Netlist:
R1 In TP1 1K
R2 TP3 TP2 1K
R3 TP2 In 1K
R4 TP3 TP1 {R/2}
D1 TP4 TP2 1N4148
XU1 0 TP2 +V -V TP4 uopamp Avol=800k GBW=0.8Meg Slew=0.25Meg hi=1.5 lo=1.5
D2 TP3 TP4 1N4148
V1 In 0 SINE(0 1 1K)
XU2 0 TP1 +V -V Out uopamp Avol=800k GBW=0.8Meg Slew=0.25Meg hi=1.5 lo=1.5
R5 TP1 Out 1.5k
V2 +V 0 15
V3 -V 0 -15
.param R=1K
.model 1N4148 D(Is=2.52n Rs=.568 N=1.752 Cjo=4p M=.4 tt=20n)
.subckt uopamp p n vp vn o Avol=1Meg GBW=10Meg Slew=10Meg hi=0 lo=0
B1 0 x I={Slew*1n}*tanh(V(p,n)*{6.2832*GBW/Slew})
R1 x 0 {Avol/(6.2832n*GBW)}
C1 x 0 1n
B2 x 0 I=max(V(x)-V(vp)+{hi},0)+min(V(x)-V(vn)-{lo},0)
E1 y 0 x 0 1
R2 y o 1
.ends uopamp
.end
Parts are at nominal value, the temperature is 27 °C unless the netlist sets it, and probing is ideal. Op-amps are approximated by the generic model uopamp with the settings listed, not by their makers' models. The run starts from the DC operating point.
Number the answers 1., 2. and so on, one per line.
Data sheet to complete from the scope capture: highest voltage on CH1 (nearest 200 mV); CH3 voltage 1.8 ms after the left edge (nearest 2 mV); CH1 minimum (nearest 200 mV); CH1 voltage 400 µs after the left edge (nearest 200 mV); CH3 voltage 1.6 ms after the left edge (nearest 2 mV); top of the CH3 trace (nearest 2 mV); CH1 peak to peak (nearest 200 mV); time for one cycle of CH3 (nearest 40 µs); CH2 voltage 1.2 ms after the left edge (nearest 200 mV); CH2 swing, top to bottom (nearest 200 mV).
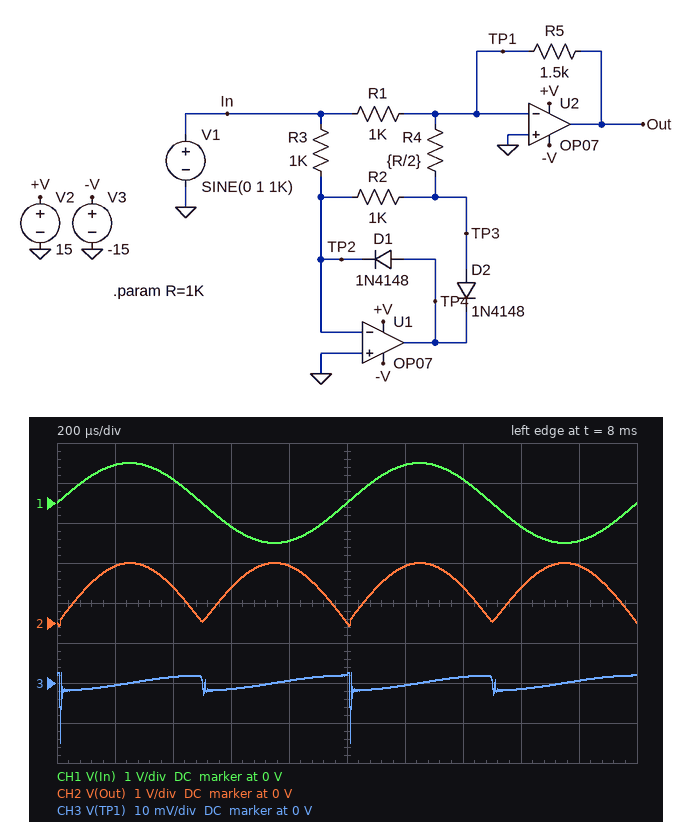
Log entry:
1. 1.0 V
2. 0 V
3. -1.0 V
4. 600 mV
5. -2 mV
6. 2 mV
7. 2.0 V
8. 1.00 ms
9. 1.4 V
10. 1.6 V
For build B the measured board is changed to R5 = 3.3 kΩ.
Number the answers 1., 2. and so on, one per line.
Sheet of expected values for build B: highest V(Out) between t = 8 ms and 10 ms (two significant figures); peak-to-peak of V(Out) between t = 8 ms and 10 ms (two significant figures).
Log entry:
1. 3.3 V
2. 3.5 V
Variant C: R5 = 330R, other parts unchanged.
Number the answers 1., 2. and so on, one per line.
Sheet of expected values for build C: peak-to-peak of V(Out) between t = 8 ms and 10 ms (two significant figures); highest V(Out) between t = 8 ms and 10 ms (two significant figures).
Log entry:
1. 350 mV
2. 330 mV
